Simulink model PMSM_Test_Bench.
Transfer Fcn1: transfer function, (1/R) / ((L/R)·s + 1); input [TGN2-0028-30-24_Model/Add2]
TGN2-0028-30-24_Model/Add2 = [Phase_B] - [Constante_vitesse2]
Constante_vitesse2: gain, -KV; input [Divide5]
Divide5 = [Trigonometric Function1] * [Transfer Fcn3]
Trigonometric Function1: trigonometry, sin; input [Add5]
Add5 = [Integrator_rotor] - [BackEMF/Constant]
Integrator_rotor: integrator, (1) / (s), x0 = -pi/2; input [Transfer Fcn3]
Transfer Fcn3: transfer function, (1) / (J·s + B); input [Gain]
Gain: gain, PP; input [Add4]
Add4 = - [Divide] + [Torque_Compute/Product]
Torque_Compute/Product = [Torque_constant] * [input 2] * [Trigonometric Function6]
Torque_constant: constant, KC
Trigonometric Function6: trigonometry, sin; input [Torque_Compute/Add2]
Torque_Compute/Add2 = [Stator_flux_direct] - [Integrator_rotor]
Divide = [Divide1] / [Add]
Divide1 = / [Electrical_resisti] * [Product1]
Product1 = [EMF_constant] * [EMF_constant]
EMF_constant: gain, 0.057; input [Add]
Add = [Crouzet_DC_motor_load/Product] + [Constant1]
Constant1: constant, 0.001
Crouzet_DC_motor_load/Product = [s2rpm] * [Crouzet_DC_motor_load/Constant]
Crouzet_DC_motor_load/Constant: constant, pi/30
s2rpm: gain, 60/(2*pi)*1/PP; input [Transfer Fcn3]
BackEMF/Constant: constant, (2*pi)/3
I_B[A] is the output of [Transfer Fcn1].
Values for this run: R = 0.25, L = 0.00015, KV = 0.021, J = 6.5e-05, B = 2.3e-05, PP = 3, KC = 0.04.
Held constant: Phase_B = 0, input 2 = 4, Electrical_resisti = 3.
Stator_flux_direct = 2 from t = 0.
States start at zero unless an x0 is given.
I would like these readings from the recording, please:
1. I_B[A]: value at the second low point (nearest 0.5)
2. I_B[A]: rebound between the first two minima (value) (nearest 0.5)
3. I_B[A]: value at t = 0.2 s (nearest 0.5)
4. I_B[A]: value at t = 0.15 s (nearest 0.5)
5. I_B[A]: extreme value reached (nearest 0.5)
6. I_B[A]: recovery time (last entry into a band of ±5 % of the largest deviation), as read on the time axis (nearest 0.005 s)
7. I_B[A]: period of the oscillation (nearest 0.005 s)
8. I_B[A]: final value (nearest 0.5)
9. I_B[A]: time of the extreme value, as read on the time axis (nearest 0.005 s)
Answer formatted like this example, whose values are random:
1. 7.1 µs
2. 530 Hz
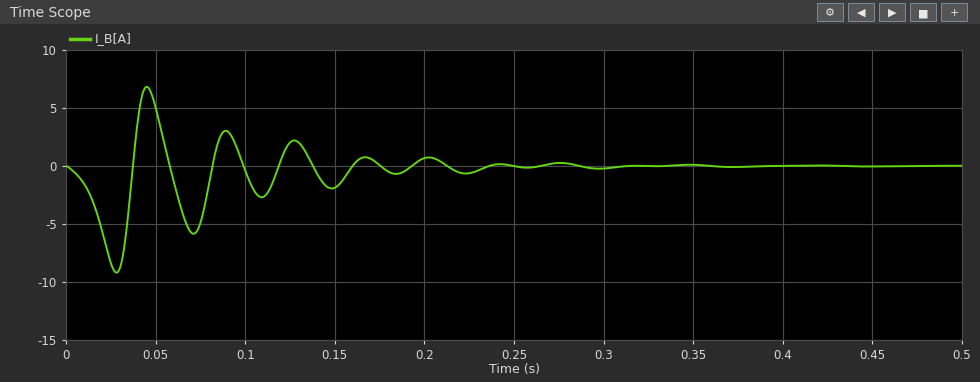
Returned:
1. -6.0
2. 7.0
3. 0.5
4. -2.0
5. -9.0
6. 0.230 s
7. 0.045 s
8. 0.0
9. 0.030 s
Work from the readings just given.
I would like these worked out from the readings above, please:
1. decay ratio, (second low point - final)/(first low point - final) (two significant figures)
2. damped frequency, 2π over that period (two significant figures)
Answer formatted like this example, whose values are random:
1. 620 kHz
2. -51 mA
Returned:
1. 0.67
2. 140 rad/s
